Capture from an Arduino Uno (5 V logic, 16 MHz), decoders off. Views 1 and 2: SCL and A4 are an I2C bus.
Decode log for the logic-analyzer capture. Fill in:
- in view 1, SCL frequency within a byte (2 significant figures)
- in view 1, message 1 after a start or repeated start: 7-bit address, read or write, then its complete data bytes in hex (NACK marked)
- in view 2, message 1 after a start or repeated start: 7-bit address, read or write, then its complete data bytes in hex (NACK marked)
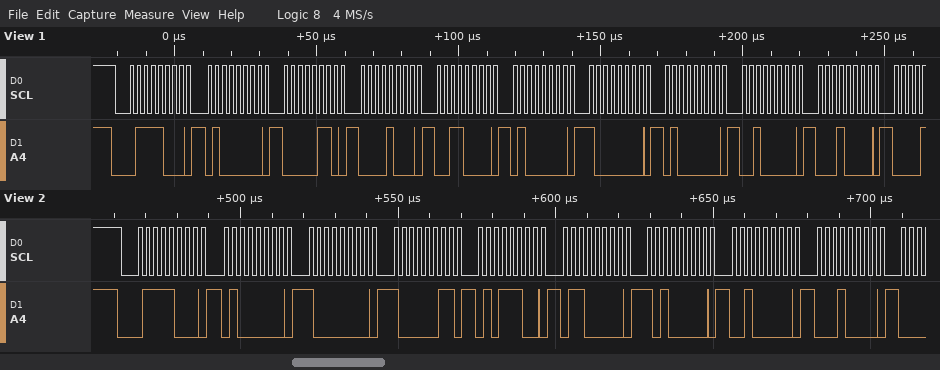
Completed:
400 kHz
0x3C write: 40 06 08 30 40 80 40 20 10
0x3C write: 40 80 83 5C 60 A0 20 10
